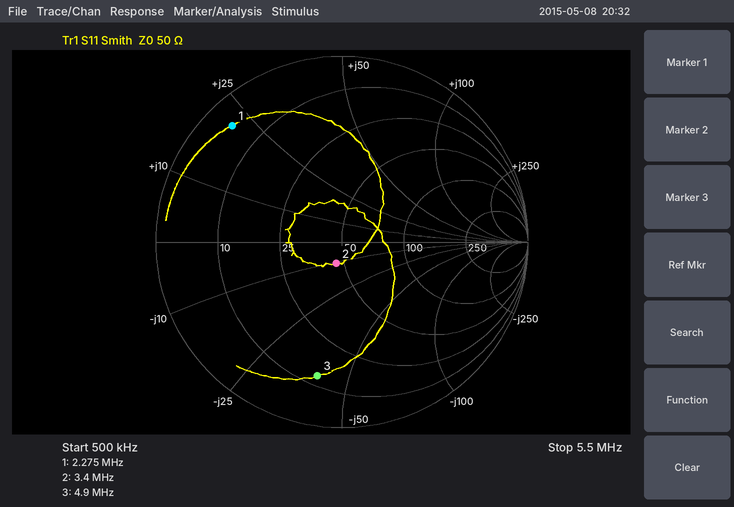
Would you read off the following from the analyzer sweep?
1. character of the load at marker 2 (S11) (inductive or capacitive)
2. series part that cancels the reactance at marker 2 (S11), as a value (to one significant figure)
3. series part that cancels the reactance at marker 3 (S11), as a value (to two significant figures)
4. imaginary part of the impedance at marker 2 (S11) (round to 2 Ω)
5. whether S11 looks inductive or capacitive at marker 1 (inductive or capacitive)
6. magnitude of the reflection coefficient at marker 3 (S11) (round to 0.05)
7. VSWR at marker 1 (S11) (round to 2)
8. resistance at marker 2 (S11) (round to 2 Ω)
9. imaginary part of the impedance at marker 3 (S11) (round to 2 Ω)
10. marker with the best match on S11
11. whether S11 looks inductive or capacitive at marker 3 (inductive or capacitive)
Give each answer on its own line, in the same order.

capacitive
500 nH
1.3 µH
-10 Ω
inductive
0.75
14
46 Ω
-40 Ω
marker 2
capacitive
